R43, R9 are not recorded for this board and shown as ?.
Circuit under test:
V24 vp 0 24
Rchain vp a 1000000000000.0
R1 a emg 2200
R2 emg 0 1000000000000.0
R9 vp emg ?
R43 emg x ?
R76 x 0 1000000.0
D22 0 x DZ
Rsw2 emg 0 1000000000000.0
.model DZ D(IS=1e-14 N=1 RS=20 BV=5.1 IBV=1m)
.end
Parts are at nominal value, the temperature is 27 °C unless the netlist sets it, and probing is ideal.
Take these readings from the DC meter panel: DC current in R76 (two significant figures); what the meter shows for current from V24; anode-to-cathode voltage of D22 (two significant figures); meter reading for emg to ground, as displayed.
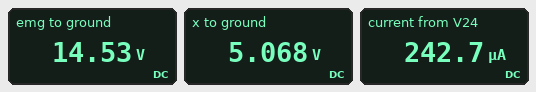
5.1 µA
242.7 µA
-5.1 V
14.53 V
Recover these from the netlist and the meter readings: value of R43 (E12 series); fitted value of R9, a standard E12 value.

39 kΩ
39 kΩ
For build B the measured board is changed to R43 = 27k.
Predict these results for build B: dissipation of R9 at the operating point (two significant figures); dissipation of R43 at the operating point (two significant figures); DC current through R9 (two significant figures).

3.2 mW
2.2 mW
290 µA
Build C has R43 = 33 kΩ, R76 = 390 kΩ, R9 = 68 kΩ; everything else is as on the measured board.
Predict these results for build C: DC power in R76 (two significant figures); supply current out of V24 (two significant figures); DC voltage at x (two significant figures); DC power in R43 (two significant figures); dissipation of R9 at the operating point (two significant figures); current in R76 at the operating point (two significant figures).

66 µW
190 µA
5.1 V
1.2 mW
2.4 mW
13 µA
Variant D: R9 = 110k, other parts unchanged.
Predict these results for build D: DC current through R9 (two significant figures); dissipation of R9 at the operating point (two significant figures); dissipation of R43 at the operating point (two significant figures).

130 µA
1.8 mW
630 µW
